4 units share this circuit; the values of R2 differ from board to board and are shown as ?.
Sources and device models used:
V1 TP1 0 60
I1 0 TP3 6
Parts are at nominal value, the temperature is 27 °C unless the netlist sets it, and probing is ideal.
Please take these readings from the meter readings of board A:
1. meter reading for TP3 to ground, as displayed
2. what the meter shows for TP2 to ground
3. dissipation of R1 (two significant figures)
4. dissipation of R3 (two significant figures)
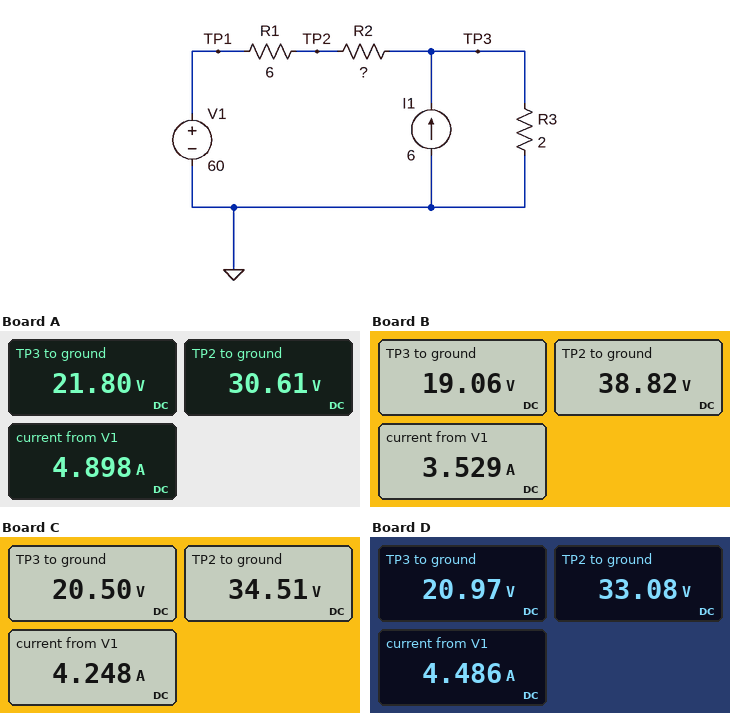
21.80 V
30.61 V
140 W
240 W
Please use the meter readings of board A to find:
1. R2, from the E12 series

1.8 Ω
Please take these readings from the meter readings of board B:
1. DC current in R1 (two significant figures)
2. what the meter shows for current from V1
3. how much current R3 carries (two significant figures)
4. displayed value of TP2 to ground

3.5 A
3.529 A
9.5 A
38.82 V
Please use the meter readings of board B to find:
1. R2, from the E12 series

5.6 Ω
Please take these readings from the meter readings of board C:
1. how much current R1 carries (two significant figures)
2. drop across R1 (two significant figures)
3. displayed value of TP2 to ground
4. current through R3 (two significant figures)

4.2 A
25 V
34.51 V
10 A
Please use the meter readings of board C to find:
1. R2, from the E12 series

3.3 Ω
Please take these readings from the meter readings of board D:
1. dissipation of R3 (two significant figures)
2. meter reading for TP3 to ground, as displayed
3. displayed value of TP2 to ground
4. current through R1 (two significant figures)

220 W
20.97 V
33.08 V
4.5 A
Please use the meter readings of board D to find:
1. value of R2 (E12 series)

2.7 Ω
